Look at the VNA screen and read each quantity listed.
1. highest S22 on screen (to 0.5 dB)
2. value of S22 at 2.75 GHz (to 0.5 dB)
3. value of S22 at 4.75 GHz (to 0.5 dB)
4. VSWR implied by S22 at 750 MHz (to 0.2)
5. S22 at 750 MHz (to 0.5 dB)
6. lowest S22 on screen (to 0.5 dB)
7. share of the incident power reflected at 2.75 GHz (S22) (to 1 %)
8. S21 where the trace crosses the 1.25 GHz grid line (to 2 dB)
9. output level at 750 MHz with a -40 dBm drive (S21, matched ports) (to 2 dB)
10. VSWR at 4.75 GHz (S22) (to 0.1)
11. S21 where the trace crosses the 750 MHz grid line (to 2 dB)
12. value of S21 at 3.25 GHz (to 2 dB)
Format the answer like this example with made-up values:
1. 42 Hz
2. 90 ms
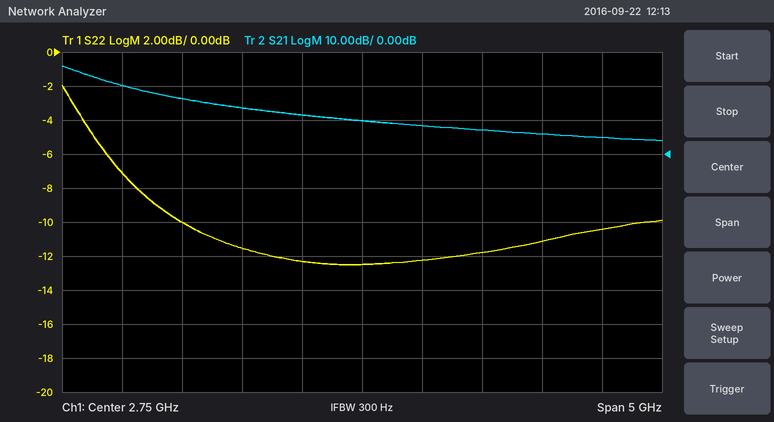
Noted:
1. -2.0 dB
2. -12.5 dB
3. -10.5 dB
4. 2.6
5. -7.0 dB
6. -12.5 dB
7. 6 %
8. 16 dB
9. -20 dBm
10. 1.9
11. 20 dB
12. 8 dB
